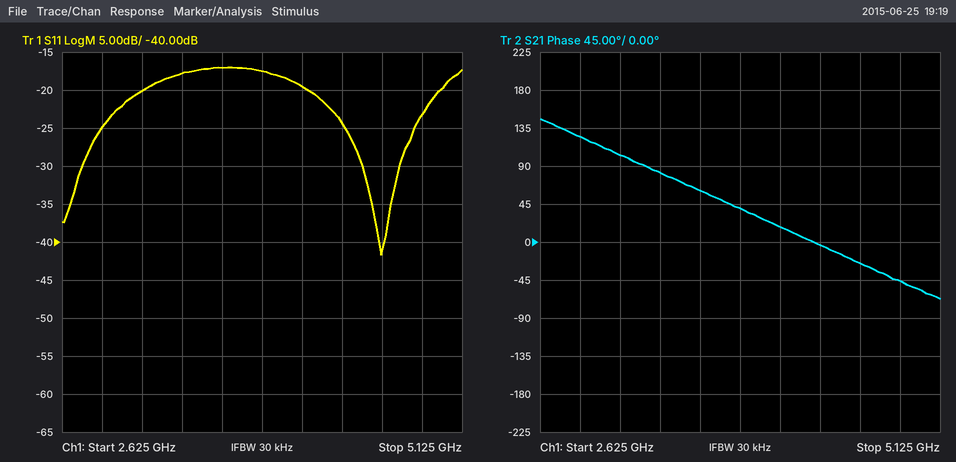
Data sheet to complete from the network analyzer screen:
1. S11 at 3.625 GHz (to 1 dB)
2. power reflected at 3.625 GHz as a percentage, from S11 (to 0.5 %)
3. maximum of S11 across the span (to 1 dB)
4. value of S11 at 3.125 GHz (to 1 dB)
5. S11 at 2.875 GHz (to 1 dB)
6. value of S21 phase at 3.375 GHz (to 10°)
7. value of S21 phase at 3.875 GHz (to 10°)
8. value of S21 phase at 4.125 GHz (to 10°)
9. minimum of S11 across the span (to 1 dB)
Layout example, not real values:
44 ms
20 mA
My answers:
-17 dB
2.0 %
-17 dB
-20 dB
-25 dB
80°
40°
20°
-42 dB
